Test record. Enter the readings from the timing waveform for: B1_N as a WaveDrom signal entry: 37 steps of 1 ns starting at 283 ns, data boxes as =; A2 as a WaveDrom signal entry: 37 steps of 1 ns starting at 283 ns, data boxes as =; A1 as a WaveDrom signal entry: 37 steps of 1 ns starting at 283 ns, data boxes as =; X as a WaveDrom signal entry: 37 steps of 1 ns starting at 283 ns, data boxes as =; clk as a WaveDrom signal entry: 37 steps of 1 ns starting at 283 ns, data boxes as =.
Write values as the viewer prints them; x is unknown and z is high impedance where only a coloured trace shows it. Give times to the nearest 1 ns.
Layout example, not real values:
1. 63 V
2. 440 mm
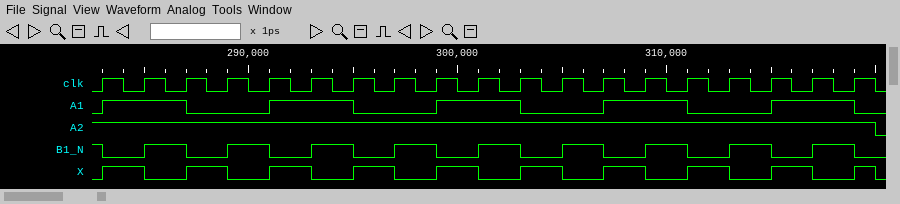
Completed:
1. {name: 'B1_N', wave: '0.1.0.1.0.1.0.1.0.1.0.1.0.1.0.1.0.1.0'}
2. {name: 'A2', wave: '1....................................'}
3. {name: 'A1', wave: '1...0...1...0...1...0...1...0...1...0'}
4. {name: 'X', wave: '1.0.1.0.1.0.1.0.1.0.1.0.1.0.1.0.1.0.1'}
5. {name: 'clk', wave: '1010101010101010101010101010101010101'}
